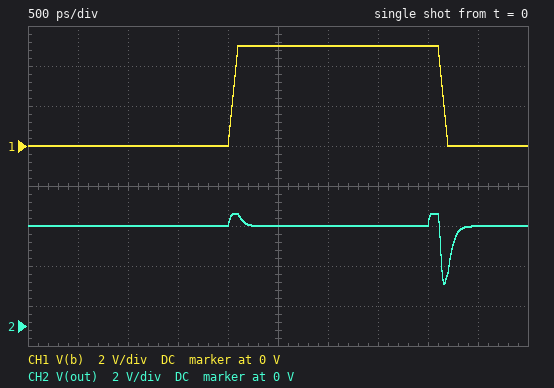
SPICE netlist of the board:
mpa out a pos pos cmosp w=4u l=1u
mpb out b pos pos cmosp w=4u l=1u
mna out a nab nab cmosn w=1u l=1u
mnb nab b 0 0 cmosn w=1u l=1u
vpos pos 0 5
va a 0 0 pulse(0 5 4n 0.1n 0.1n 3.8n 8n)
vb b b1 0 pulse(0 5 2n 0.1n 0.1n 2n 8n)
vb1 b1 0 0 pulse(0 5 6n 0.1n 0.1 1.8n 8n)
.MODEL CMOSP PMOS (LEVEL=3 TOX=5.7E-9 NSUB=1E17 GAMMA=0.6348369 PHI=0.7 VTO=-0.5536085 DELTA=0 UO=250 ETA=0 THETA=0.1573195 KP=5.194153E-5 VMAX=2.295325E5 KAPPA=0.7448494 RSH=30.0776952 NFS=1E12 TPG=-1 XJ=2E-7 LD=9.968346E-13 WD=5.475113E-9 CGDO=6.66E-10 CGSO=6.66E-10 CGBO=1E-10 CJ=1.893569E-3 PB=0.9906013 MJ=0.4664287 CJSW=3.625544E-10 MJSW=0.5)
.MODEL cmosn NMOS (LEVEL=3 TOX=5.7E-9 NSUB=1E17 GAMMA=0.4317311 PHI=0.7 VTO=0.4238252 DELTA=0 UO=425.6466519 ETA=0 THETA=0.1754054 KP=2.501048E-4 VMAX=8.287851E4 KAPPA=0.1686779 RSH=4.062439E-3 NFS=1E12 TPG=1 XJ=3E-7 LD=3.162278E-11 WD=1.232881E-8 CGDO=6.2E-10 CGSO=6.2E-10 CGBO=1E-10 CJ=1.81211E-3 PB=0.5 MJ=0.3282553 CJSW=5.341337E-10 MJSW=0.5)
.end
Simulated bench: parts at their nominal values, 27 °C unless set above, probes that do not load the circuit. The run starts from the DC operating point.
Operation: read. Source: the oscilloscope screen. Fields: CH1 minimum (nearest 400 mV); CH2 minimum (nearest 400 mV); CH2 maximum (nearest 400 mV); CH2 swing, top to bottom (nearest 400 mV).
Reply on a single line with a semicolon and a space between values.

0 V; 2.0 V; 5.6 V; 3.6 V
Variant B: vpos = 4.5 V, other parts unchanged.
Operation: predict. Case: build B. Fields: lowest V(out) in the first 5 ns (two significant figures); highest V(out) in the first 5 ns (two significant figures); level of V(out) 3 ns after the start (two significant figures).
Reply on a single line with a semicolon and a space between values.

1.1 V; 5.1 V; 4.5 V
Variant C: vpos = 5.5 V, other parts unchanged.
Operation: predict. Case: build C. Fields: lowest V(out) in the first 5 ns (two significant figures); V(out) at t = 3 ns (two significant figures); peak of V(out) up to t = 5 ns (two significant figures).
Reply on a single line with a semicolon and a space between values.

3.2 V; 5.5 V; 6.1 V
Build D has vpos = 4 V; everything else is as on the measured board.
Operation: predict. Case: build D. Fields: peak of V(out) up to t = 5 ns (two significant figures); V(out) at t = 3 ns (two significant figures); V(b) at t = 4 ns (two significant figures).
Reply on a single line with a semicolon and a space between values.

4.6 V; 4.0 V; 5.0 V
